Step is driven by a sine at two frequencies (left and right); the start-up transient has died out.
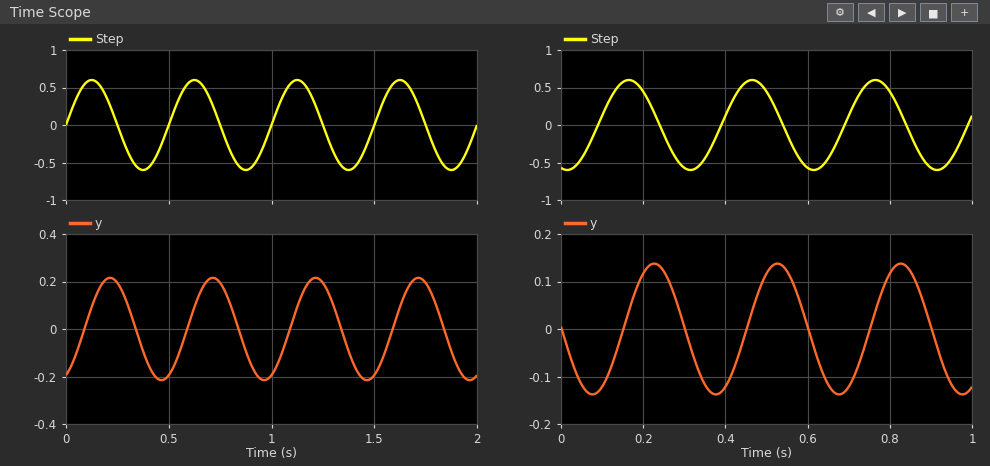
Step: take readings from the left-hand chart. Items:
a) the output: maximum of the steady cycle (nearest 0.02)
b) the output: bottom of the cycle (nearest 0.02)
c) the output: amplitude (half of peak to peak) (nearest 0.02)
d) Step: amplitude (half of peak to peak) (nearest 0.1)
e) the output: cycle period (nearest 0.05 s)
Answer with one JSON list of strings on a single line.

["0.22", "-0.22", "0.22", "0.6", "0.50 s"]
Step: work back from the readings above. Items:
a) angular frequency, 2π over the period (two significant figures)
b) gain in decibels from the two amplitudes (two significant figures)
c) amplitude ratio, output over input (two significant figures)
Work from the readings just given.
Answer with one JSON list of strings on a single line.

["13 rad/s", "-8.7 dB", "0.37"]
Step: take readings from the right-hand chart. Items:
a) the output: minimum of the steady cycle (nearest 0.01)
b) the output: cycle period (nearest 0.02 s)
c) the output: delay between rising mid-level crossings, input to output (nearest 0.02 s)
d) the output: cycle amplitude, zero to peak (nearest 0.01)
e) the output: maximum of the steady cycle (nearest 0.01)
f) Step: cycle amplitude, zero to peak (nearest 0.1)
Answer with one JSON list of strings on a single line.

["-0.14", "0.30 s", "0.06 s", "0.14", "0.14", "0.6"]
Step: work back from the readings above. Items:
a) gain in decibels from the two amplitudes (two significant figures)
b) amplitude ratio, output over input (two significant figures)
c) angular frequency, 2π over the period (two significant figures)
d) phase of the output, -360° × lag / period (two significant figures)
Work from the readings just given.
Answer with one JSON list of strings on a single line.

["-13 dB", "0.23", "21 rad/s", "-72°"]
